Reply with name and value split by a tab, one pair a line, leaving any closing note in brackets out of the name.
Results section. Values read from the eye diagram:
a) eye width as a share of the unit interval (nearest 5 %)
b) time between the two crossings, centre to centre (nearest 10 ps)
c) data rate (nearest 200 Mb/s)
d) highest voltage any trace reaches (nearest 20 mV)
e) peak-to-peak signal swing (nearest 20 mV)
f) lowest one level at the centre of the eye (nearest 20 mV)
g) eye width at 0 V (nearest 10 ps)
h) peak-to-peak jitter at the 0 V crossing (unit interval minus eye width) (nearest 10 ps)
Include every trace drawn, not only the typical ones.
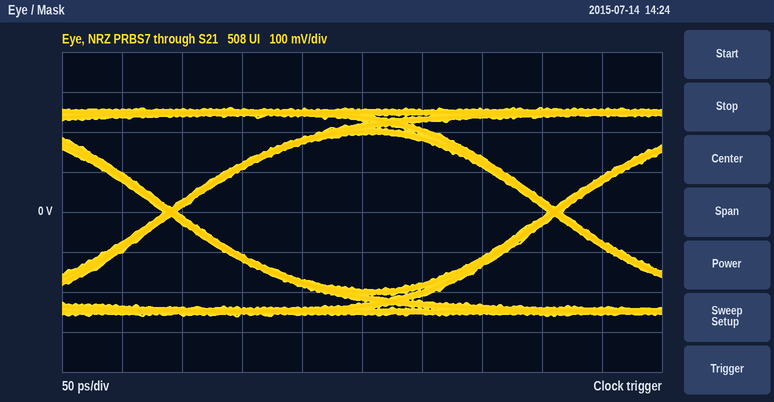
eye width as a share of the unit interval	95 %
time between the two crossings, centre to centre	320 ps
data rate	3.2 Gb/s
highest voltage any trace reaches	260 mV
peak-to-peak signal swing	520 mV
lowest one level at the centre of the eye	200 mV
eye width at 0 V	310 ps
peak-to-peak jitter at the 0 V crossing (unit interval minus eye width)	10 ps
